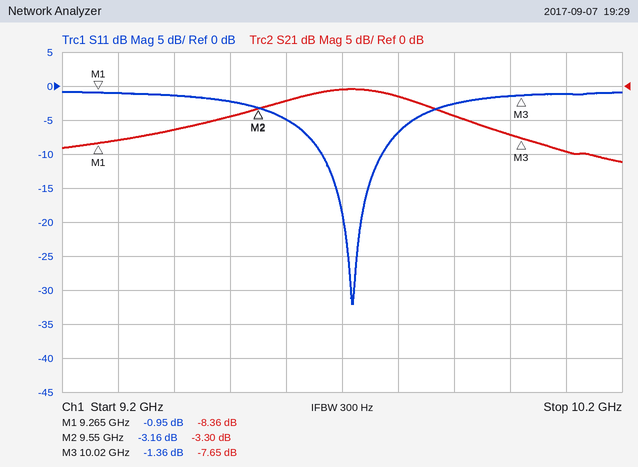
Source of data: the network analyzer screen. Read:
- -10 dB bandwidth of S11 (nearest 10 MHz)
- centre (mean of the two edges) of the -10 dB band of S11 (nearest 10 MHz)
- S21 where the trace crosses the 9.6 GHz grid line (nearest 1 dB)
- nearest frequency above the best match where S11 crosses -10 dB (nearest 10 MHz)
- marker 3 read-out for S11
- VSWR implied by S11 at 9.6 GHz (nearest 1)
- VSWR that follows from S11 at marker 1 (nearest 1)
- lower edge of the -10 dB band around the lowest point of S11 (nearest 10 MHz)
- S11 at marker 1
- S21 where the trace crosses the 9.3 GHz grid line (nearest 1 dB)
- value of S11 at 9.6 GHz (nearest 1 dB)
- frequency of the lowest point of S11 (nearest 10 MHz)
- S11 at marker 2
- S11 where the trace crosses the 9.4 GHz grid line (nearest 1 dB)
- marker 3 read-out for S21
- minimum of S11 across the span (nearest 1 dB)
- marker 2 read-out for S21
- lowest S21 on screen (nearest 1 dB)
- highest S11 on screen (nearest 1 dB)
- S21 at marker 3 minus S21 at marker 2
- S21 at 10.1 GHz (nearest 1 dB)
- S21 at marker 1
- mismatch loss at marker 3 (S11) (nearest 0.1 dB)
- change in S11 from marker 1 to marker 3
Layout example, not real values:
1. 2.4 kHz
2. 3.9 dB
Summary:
1. 110 MHz
2. 9.72 GHz
3. -2 dB
4. 9.77 GHz
5. -1.36 dB
6. 4
7. 18
8. 9.66 GHz
9. -0.95 dB
10. -8 dB
11. -5 dB
12. 9.72 GHz
13. -3.16 dB
14. -1 dB
15. -7.65 dB
16. -32 dB
17. -3.30 dB
18. -11 dB
19. -1 dB
20. -4.35 dB
21. -10 dB
22. -8.36 dB
23. 5.7 dB
24. -0.41 dB
